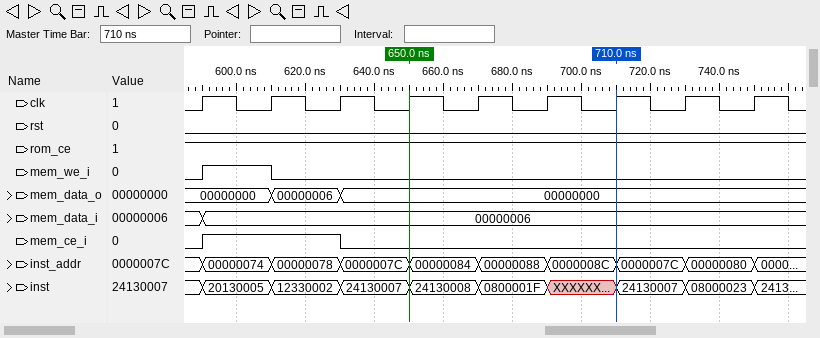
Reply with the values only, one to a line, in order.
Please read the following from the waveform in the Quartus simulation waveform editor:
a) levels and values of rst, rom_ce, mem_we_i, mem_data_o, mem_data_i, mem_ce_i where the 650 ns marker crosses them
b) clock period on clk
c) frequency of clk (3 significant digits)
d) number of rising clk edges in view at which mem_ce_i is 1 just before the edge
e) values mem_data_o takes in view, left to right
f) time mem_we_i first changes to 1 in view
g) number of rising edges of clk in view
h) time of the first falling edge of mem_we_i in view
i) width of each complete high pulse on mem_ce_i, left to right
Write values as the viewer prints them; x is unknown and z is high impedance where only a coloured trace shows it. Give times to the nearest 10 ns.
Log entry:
rst=0, rom_ce=1, mem_we_i=0, mem_data_o=00000000, mem_data_i=00000006, mem_ce_i=0
20 ns
50.0 MHz
2
00000000, 00000006, 00000000
590 ns
9
610 ns
40 ns
